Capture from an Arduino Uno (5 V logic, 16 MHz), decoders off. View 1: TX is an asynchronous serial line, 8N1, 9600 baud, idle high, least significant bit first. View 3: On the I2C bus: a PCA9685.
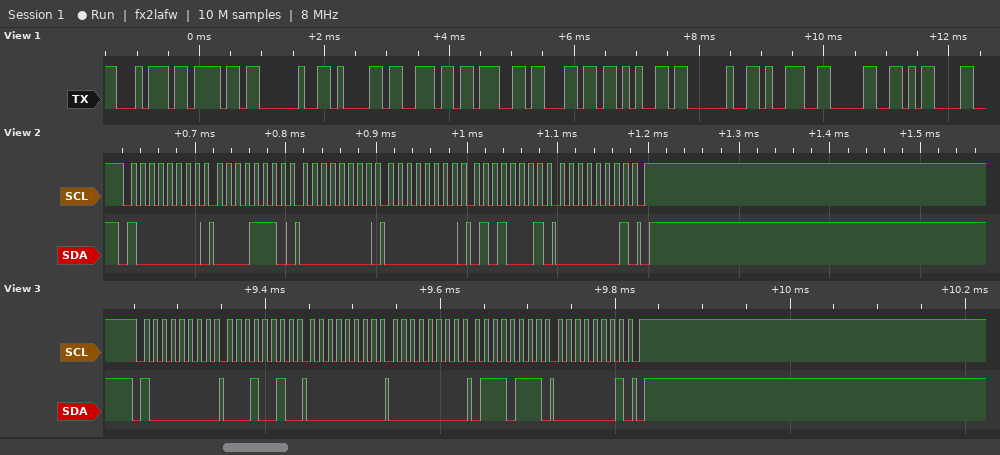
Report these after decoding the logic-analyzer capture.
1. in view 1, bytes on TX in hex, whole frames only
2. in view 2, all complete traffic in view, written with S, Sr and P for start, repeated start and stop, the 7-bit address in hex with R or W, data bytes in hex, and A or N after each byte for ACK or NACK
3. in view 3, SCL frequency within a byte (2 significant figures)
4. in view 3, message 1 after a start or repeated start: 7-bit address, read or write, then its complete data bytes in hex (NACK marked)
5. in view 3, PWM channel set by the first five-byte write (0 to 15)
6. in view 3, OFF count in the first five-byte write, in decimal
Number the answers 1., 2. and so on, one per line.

1. 74 6F 20 61 6E 67 6C 65 20 39 30 0D
2. S 40W A 0E A 00 A 00 A 51 A 01 A P
3. 100 kHz
4. 0x40 write: 12 00 00 77 01
5. 3
6. 375
